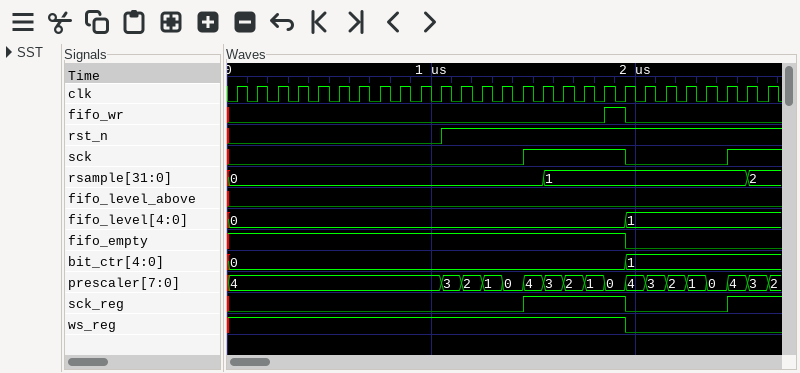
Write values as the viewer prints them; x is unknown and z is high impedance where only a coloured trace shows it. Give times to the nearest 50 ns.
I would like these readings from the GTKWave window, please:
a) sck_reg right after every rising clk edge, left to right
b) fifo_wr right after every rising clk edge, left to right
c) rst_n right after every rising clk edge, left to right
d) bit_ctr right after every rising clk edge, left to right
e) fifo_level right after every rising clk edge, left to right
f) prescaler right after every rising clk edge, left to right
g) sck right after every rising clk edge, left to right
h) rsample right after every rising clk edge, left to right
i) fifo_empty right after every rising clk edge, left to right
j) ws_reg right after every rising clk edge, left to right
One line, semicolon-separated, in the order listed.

0 0 0 0 0 0 0 0 0 0 0 0 0 0 1 1 1 1 1 0 0 0 0 0 1 1 1; 0 0 0 0 0 0 0 0 0 0 0 0 0 0 0 0 0 0 1 0 0 0 0 0 0 0 0; 0 0 0 0 0 0 0 0 0 0 1 1 1 1 1 1 1 1 1 1 1 1 1 1 1 1 1; 0, 0, 0, 0, 0, 0, 0, 0, 0, 0, 0, 0, 0, 0, 0, 0, 0, 0, 0, 1, 1, 1, 1, 1, 1, 1, 1; 0, 0, 0, 0, 0, 0, 0, 0, 0, 0, 0, 0, 0, 0, 0, 0, 0, 0, 0, 1, 1, 1, 1, 1, 1, 1, 1; 4, 4, 4, 4, 4, 4, 4, 4, 4, 4, 3, 2, 1, 0, 4, 3, 2, 1, 0, 4, 3, 2, 1, 0, 4, 3, 2; 0 0 0 0 0 0 0 0 0 0 0 0 0 0 1 1 1 1 1 0 0 0 0 0 1 1 1; 0, 0, 0, 0, 0, 0, 0, 0, 0, 0, 0, 0, 0, 0, 0, 1, 1, 1, 1, 1, 1, 1, 1, 1, 1, 2, 2; 1 1 1 1 1 1 1 1 1 1 1 1 1 1 1 1 1 1 1 0 0 0 0 0 0 0 0; 1 1 1 1 1 1 1 1 1 1 1 1 1 1 1 1 1 1 1 0 0 0 0 0 0 0 0
